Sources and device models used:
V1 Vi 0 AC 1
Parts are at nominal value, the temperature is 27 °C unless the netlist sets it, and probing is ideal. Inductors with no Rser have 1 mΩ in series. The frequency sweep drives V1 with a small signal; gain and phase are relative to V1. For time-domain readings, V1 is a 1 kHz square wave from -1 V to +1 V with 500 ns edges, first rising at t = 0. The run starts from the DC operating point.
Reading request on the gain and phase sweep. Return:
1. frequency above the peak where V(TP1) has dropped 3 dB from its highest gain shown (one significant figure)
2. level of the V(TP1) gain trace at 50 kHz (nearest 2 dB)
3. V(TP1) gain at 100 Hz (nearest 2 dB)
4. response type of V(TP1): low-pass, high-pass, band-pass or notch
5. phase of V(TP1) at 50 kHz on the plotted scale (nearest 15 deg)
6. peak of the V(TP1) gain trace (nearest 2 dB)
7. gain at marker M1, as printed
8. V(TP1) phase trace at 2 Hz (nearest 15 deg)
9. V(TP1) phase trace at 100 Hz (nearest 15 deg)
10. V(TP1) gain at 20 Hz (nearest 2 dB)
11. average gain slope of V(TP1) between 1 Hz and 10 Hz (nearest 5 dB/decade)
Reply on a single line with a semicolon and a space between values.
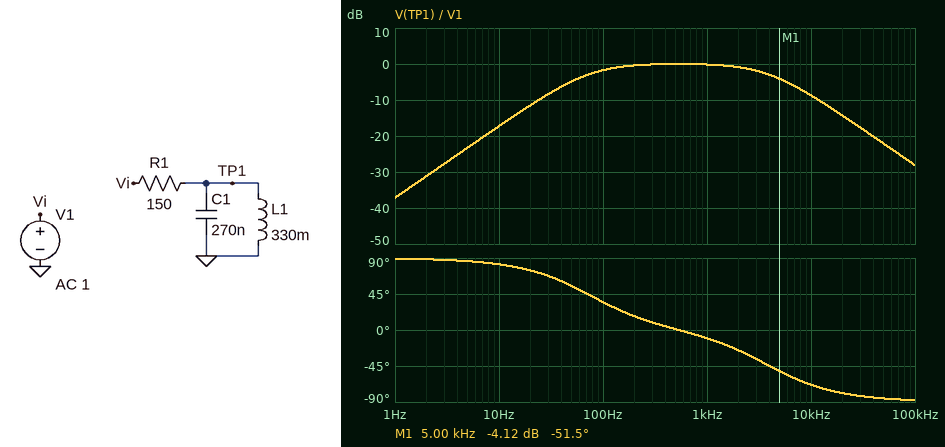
4 kHz; -22 dB; -2 dB; band-pass; -90 deg; 0 dB; -4.12 dB; 90 deg; 30 deg; -12 dB; 20 dB/decade
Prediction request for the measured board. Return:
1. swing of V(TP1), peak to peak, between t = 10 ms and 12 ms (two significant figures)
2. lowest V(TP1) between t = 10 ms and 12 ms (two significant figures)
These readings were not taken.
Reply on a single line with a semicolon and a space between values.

2.1 V; -1.0 V
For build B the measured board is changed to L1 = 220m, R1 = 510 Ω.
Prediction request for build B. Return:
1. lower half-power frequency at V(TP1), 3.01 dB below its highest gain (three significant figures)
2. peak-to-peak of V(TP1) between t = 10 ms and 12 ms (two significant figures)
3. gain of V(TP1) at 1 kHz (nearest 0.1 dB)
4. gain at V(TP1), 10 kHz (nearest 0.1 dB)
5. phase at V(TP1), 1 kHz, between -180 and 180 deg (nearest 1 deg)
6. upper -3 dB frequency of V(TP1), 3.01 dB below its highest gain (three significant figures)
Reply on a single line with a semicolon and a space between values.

294 Hz; 2.0 V; -1.0 dB; -18.8 dB; -26 deg; 1.45 kHz
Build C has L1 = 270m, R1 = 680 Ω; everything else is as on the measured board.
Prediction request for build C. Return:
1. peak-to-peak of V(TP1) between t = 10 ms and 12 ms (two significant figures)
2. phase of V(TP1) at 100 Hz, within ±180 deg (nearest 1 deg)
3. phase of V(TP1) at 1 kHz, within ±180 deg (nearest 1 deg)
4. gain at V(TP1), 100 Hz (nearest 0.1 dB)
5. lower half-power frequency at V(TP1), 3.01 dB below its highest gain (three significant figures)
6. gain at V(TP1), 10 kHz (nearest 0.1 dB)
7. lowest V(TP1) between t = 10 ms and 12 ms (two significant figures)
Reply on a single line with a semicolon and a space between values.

1.9 V; 76 deg; -37 deg; -12.1 dB; 298 Hz; -21.2 dB; -930 mV
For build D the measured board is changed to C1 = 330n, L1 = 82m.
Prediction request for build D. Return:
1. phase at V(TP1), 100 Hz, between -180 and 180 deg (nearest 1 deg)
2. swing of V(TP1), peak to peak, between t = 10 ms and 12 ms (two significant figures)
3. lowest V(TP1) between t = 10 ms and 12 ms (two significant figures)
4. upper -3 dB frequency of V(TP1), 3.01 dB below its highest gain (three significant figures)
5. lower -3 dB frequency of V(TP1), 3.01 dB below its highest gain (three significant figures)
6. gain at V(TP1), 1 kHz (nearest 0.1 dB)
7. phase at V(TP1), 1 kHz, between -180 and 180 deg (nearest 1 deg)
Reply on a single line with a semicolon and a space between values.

71 deg; 2.4 V; -1.2 V; 3.48 kHz; 269 Hz; 0 dB; -1 deg
